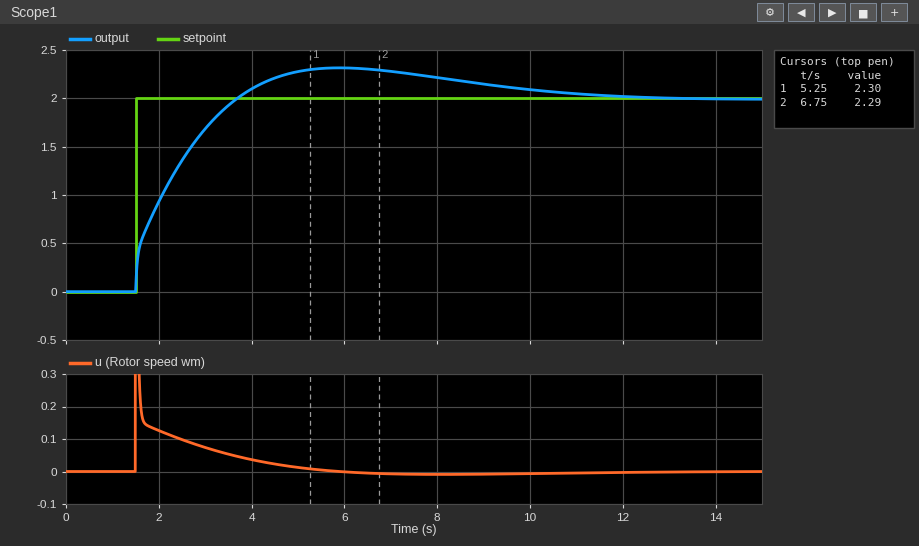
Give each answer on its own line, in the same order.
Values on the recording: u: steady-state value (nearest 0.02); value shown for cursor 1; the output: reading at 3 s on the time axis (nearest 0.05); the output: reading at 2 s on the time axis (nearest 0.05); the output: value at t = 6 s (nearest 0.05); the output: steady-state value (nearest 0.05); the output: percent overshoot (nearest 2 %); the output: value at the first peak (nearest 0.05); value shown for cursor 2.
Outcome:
0.00
2.30
1.70
0.95
2.30
2.00
16 %
2.30
2.29
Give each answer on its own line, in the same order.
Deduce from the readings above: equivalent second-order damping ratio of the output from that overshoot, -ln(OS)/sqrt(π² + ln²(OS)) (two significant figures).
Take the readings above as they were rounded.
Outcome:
0.50
